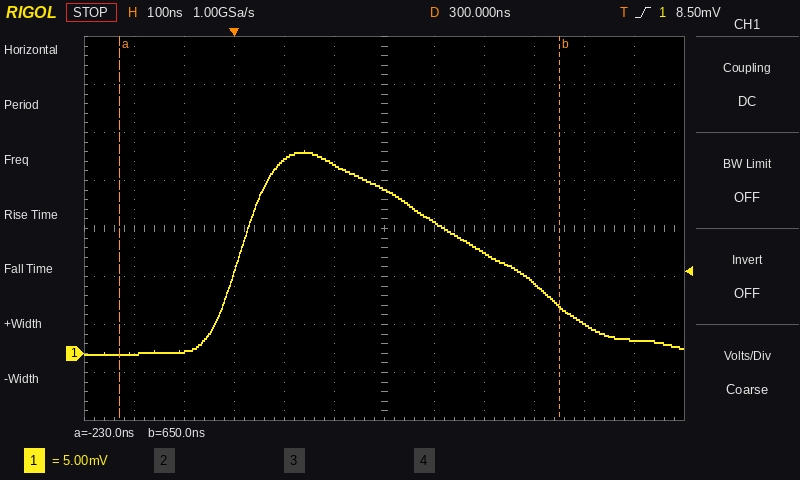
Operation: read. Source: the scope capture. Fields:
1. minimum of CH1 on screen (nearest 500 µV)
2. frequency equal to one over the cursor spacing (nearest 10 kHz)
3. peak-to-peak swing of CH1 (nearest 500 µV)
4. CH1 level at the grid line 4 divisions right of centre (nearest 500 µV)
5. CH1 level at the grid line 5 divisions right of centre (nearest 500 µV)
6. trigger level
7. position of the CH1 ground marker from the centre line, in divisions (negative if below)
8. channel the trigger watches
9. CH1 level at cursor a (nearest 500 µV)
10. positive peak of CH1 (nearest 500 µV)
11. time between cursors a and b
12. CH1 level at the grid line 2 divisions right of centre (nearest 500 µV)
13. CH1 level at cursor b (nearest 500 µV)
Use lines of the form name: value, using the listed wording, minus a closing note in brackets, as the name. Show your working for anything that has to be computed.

minimum of CH1 on screen: 0.0 mV
frequency equal to one over the cursor spacing: 1 / 880 ns ≈ 1.14 MHz
peak-to-peak swing of CH1: 21.0 mV − (0.0 mV) = 21.0 mV
CH1 level at the grid line 4 divisions right of centre: 3.0 mV
CH1 level at the grid line 5 divisions right of centre: 1.5 mV
trigger level: 8.50 mV
position of the CH1 ground marker from the centre line, in divisions: -2.6 div
channel the trigger watches: CH1
CH1 level at cursor a: 0.0 mV
positive peak of CH1: 21.0 mV
time between cursors a and b: 650 ns − (-230 ns) = 880 ns
CH1 level at the grid line 2 divisions right of centre: 10.5 mV
CH1 level at cursor b: 5.0 mV
